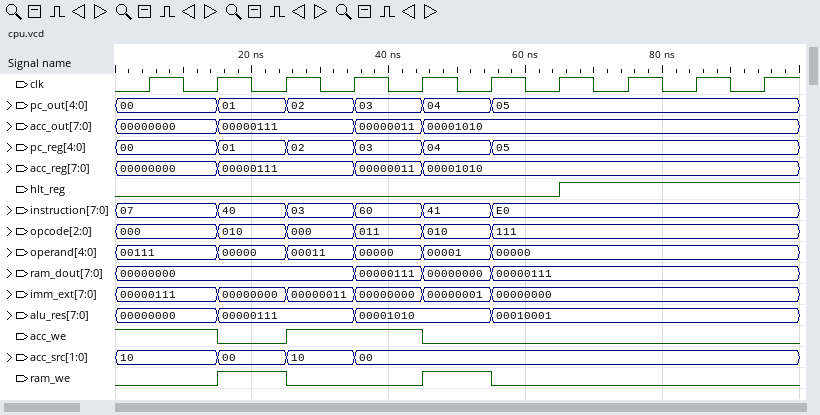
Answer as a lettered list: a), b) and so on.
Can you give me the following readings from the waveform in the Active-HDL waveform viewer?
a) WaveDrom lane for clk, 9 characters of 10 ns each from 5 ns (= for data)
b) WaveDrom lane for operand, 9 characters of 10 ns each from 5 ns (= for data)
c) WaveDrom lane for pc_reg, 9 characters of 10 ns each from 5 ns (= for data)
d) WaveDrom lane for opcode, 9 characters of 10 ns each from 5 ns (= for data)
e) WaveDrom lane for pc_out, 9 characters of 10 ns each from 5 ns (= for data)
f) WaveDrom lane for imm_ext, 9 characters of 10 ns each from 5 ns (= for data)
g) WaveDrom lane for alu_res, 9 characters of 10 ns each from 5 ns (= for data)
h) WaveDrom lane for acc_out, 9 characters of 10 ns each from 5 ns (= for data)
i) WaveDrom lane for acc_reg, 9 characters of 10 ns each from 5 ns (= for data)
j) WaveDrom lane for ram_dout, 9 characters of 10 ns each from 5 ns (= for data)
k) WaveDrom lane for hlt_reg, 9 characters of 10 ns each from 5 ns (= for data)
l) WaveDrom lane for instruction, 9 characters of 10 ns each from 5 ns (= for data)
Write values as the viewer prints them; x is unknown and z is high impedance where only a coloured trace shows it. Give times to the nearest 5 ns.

a) {name: 'clk', wave: 'p........'}
b) {name: 'operand', wave: '======...', data: '00111 00000 00011 00000 00001 00000'}
c) {name: 'pc_reg', wave: '======...', data: '00 01 02 03 04 05'}
d) {name: 'opcode', wave: '======...', data: '000 010 000 011 010 111'}
e) {name: 'pc_out', wave: '======...', data: '00 01 02 03 04 05'}
f) {name: 'imm_ext', wave: '======...', data: '00000111 00000000 00000011 00000000 00000001 00000000'}
g) {name: 'alu_res', wave: '==.=.=...', data: '00000000 00000111 00001010 00010001'}
h) {name: 'acc_out', wave: '==.==....', data: '00000000 00000111 00000011 00001010'}
i) {name: 'acc_reg', wave: '==.==....', data: '00000000 00000111 00000011 00001010'}
j) {name: 'ram_dout', wave: '=..===...', data: '00000000 00000111 00000000 00000111'}
k) {name: 'hlt_reg', wave: '0.....1..'}
l) {name: 'instruction', wave: '======...', data: '07 40 03 60 41 E0'}
